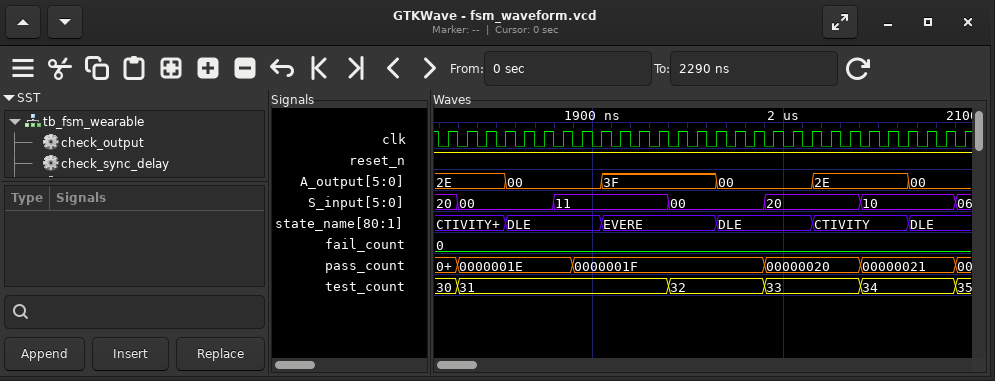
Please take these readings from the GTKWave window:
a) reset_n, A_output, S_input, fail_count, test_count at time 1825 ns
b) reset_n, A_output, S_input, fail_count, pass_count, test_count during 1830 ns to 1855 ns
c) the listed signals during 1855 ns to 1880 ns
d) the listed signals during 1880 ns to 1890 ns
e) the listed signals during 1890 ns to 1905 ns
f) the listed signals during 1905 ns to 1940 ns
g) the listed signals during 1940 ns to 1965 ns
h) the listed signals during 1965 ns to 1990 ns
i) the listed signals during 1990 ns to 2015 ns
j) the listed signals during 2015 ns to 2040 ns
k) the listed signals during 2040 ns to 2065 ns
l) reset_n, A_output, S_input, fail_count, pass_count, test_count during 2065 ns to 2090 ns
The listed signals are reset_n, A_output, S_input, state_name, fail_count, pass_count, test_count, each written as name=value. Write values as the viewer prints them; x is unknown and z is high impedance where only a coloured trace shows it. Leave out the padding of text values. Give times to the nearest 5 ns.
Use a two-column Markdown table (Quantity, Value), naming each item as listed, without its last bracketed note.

| Quantity | Value |
|---|---|
| reset_n, A_output, S_input, fail_count, test_count at time 1825 ns | reset_n=1, A_output=2E, S_input=20, fail_count=0, test_count=30 |
| reset_n, A_output, S_input, fail_count, pass_count, test_count during 1830 ns to 1855 ns | reset_n=1, A_output=2E, S_input=00, fail_count=0, pass_count=0000001E, test_count=31 |
| the listed signals during 1855 ns to 1880 ns | reset_n=1, A_output=00, S_input=00, state_name=DLE, fail_count=0, pass_count=0000001E, test_count=31 |
| the listed signals during 1880 ns to 1890 ns | reset_n=1, A_output=00, S_input=11, state_name=DLE, fail_count=0, pass_count=0000001E, test_count=31 |
| the listed signals during 1890 ns to 1905 ns | reset_n=1, A_output=00, S_input=11, state_name=DLE, fail_count=0, pass_count=0000001F, test_count=31 |
| the listed signals during 1905 ns to 1940 ns | reset_n=1, A_output=3F, S_input=11, state_name=EVERE, fail_count=0, pass_count=0000001F, test_count=31 |
| the listed signals during 1940 ns to 1965 ns | reset_n=1, A_output=3F, S_input=00, state_name=EVERE, fail_count=0, pass_count=0000001F, test_count=32 |
| the listed signals during 1965 ns to 1990 ns | reset_n=1, A_output=00, S_input=00, state_name=DLE, fail_count=0, pass_count=0000001F, test_count=32 |
| the listed signals during 1990 ns to 2015 ns | reset_n=1, A_output=00, S_input=20, state_name=DLE, fail_count=0, pass_count=00000020, test_count=33 |
| the listed signals during 2015 ns to 2040 ns | reset_n=1, A_output=2E, S_input=20, state_name=CTIVITY, fail_count=0, pass_count=00000020, test_count=33 |
| the listed signals during 2040 ns to 2065 ns | reset_n=1, A_output=2E, S_input=10, state_name=CTIVITY, fail_count=0, pass_count=00000021, test_count=34 |
| reset_n, A_output, S_input, fail_count, pass_count, test_count during 2065 ns to 2090 ns | reset_n=1, A_output=00, S_input=10, fail_count=0, pass_count=00000021, test_count=34 |
